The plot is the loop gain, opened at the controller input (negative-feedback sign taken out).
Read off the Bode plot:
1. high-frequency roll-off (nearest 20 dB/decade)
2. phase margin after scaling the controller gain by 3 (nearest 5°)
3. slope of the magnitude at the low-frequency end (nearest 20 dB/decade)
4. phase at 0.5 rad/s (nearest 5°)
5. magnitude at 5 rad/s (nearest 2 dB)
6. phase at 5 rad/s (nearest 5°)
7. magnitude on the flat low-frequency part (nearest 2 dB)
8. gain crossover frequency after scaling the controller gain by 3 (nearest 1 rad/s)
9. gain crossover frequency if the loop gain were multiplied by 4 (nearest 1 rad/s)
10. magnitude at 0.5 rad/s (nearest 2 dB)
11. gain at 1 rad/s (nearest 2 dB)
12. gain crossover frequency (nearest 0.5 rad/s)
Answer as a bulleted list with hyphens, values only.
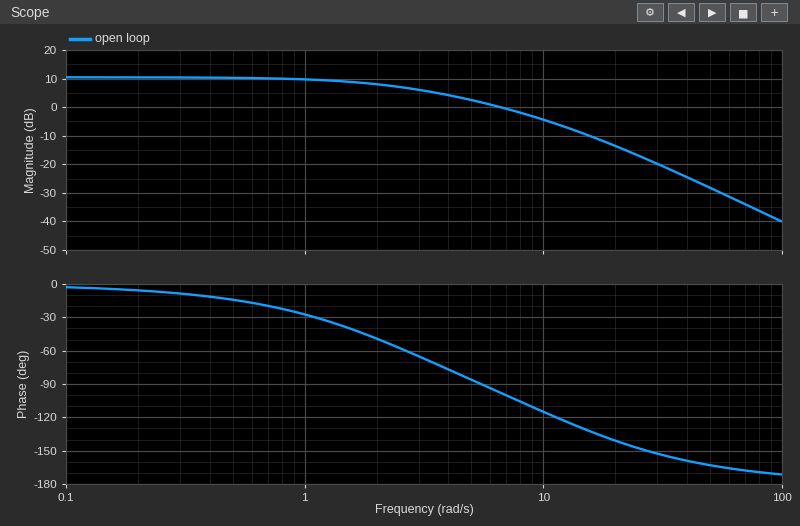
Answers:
- -40 dB/decade
- 50°
- 0 dB/decade
- -15°
- 2 dB
- -85°
- 10 dB
- 15 rad/s
- 18 rad/s
- 10 dB
- 10 dB
- 6.5 rad/s
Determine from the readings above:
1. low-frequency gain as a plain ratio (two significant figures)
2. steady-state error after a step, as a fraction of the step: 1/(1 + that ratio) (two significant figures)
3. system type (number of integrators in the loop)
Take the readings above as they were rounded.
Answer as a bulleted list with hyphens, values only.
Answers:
- 3.2
- 0.24
- 0
